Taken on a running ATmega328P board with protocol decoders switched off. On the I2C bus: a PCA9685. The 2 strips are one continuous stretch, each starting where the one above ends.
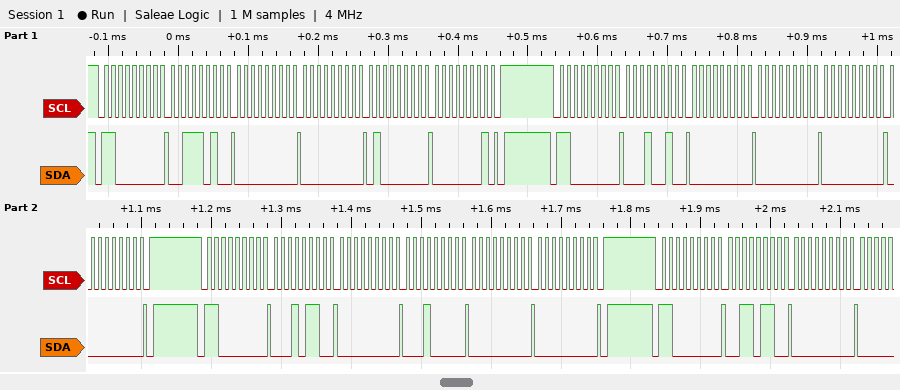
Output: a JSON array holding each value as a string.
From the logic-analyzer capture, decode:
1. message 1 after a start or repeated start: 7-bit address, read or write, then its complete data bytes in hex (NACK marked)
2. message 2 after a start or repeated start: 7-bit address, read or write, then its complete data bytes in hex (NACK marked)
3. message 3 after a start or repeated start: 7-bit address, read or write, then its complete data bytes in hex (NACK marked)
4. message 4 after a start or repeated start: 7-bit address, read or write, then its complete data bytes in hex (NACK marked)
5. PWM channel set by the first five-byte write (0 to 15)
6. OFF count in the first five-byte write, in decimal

["0x60 write: 3A 00 00 40 01", "0x60 write: 12 00 00 00 00", "0x60 write: 16 00 10 00 00", "0x60 write: 36 00", "13", "320"]
